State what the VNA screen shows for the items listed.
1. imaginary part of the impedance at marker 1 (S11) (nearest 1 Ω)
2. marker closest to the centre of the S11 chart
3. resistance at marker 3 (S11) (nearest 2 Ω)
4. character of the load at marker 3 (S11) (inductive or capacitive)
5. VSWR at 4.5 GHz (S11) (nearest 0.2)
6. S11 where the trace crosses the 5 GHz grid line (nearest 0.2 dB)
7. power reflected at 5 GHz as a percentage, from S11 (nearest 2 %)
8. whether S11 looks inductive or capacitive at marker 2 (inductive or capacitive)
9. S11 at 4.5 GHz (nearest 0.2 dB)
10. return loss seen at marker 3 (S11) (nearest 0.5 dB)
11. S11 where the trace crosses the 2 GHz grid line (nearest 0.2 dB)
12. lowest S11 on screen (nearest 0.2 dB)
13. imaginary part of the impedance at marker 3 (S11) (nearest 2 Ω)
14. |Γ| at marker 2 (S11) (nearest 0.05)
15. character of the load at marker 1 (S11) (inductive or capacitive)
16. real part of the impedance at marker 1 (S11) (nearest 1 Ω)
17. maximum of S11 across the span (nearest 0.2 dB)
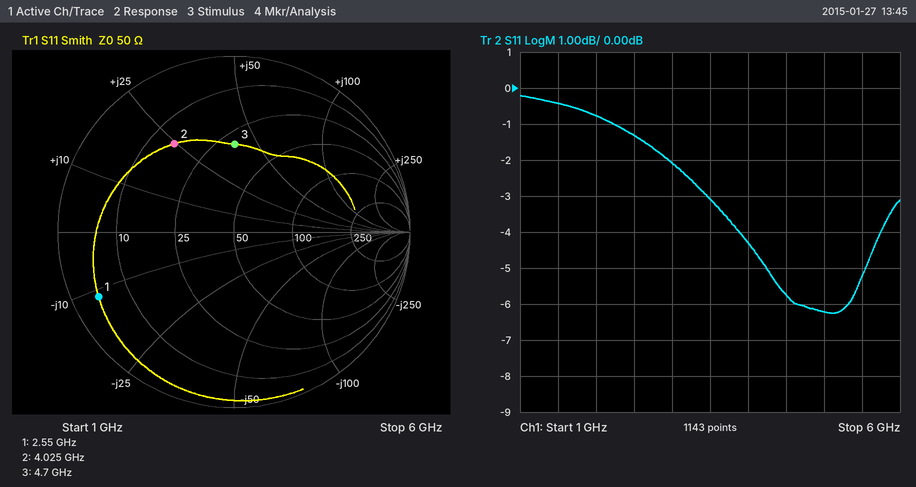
-11 Ω
marker 3
30 Ω
inductive
3.2
-6.2 dB
24 %
inductive
-5.8 dB
6.0 dB
-0.8 dB
-6.2 dB
+40 Ω
0.60
capacitive
4 Ω
-0.2 dB
